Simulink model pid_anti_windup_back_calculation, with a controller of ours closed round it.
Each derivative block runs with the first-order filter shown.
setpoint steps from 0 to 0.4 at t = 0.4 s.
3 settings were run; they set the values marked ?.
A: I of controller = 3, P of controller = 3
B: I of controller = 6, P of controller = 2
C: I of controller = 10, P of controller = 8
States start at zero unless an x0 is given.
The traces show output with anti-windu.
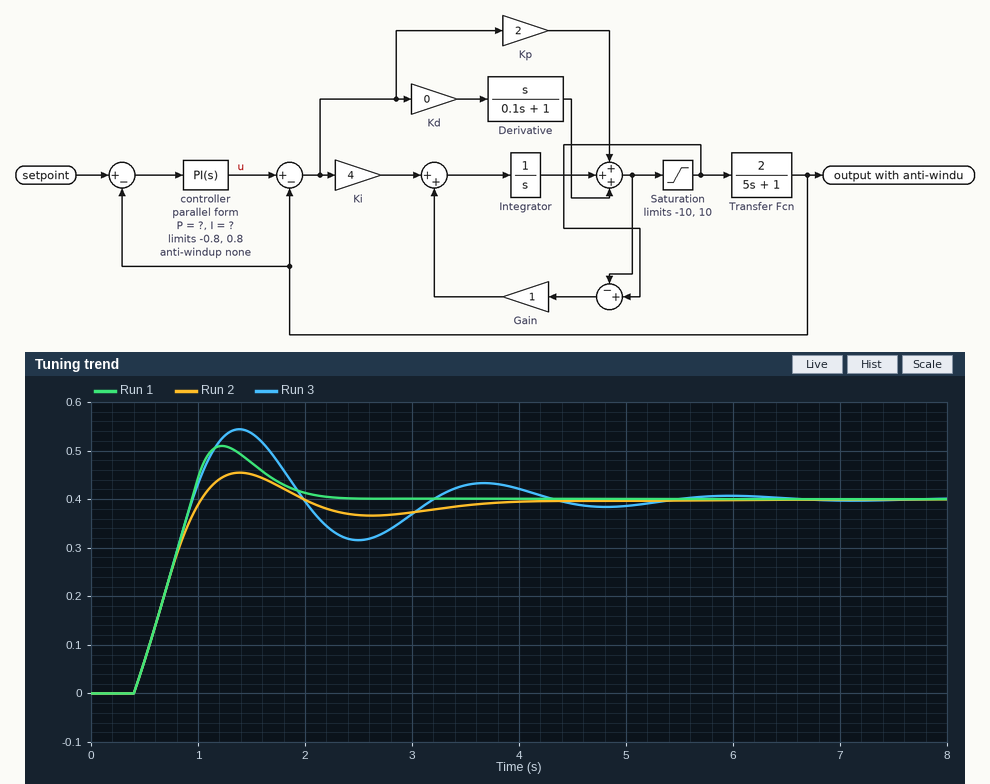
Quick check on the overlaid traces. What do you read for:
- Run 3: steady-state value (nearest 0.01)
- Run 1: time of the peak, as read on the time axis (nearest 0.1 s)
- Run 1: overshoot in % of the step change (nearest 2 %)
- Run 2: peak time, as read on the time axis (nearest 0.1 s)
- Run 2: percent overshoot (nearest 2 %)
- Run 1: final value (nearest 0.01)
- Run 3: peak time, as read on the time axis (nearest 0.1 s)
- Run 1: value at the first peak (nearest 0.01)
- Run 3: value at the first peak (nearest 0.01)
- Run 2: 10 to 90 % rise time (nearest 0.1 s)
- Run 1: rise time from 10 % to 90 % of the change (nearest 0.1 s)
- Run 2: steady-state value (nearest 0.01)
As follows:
0.40
1.2 s
28 %
1.4 s
14 %
0.40
1.4 s
0.51
0.54
0.5 s
0.4 s
0.40
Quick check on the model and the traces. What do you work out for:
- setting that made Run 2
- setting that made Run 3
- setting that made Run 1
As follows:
A
B
C
